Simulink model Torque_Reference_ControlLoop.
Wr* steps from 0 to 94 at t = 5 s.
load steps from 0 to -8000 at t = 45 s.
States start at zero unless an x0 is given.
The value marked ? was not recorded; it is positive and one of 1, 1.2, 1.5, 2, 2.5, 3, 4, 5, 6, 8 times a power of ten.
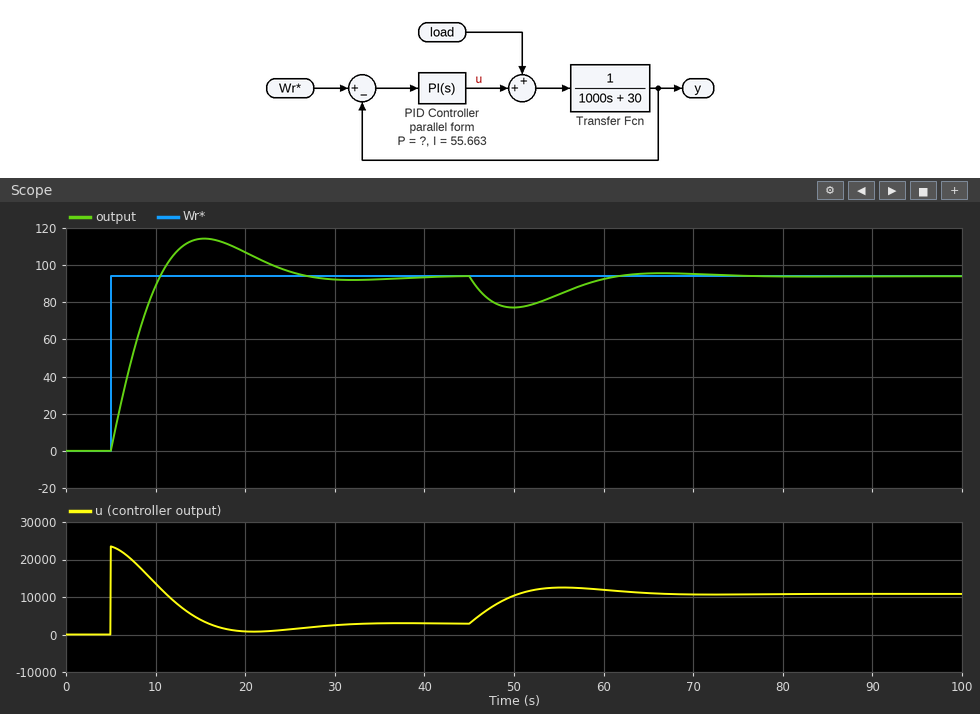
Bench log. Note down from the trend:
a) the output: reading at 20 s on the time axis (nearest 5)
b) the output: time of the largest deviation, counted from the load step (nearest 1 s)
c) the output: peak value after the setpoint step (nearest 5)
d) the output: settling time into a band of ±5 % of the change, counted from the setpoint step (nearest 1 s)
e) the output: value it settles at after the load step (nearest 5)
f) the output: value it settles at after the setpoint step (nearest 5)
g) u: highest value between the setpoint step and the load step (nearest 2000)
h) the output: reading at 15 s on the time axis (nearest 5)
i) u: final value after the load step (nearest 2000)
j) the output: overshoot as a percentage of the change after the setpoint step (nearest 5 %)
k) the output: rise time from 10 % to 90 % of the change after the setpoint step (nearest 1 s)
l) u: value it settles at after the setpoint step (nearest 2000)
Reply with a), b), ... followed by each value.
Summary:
a) 105
b) 5 s
c) 115
d) 19 s
e) 95
f) 95
g) 24000
h) 115
i) 10000
j) 20 %
k) 4 s
l) 2000
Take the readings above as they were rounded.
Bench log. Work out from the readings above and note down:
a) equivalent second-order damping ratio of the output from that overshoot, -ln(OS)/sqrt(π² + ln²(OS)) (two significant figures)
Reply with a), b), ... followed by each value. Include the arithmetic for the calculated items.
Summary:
a) ln(0.2) = -1.609; 1.609 / sqrt(9.870 + 2.590) = 0.46
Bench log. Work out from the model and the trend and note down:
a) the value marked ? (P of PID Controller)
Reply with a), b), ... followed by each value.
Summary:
a) 250
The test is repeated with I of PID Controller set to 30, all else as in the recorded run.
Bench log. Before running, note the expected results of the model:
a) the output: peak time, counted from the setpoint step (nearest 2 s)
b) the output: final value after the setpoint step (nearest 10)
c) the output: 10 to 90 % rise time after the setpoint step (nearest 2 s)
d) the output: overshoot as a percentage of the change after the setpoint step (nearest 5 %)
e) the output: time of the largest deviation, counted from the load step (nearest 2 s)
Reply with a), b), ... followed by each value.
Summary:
a) 14 s
b) 90
c) 6 s
d) 15 %
e) 6 s
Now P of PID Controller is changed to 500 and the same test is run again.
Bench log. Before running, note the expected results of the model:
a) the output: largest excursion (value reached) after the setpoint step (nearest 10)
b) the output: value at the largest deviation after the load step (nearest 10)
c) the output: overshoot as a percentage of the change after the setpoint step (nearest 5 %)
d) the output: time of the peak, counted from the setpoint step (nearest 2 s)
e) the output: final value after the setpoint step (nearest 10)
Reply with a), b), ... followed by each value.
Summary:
a) 100
b) 80
c) 10 %
d) 8 s
e) 90
